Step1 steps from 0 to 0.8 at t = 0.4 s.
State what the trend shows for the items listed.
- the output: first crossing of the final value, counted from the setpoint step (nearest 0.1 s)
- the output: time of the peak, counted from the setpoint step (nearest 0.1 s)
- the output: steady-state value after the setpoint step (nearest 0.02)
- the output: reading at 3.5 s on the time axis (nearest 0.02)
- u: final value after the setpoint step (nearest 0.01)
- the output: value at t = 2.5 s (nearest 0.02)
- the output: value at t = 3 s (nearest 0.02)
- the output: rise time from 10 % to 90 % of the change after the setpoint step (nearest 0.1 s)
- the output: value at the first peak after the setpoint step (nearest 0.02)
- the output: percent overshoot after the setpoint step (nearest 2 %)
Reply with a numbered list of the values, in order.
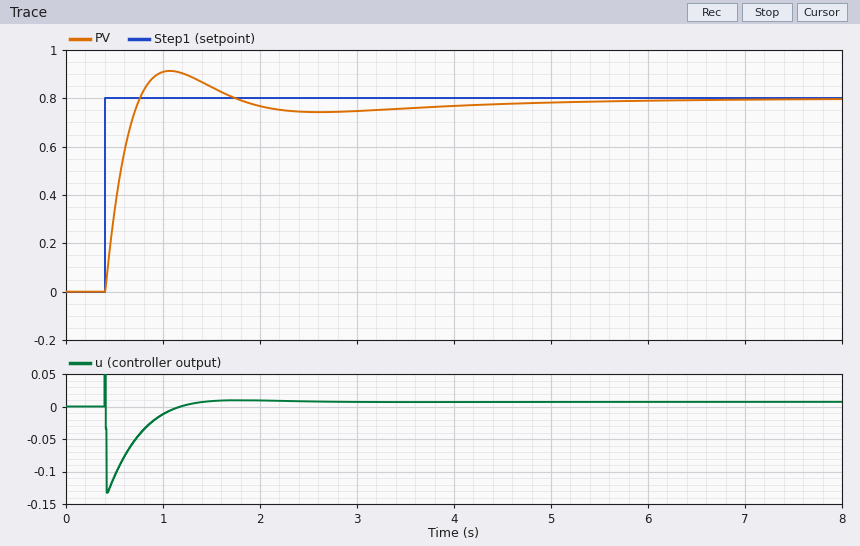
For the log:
1. 0.4 s
2. 0.7 s
3. 0.80
4. 0.76
5. 0.01
6. 0.74
7. 0.74
8. 0.3 s
9. 0.92
10. 14 %
